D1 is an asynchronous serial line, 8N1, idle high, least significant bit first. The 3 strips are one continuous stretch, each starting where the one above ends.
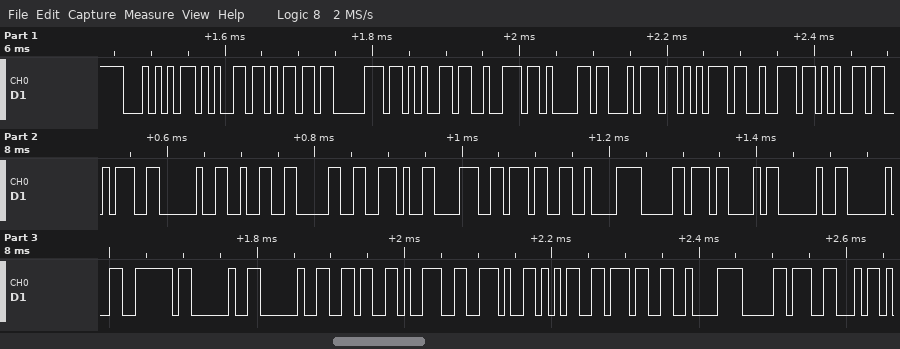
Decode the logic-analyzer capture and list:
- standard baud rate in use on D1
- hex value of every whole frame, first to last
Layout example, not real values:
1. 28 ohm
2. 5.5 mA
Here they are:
1. 115200 baud
2. 54 65 6D 70 65 72 61 74 75 72 65 3A 20 32 30 2E 38 37 C2 B0 43 20 20 7E 20 20 36 39 2E 35 37 C2 B0 46
